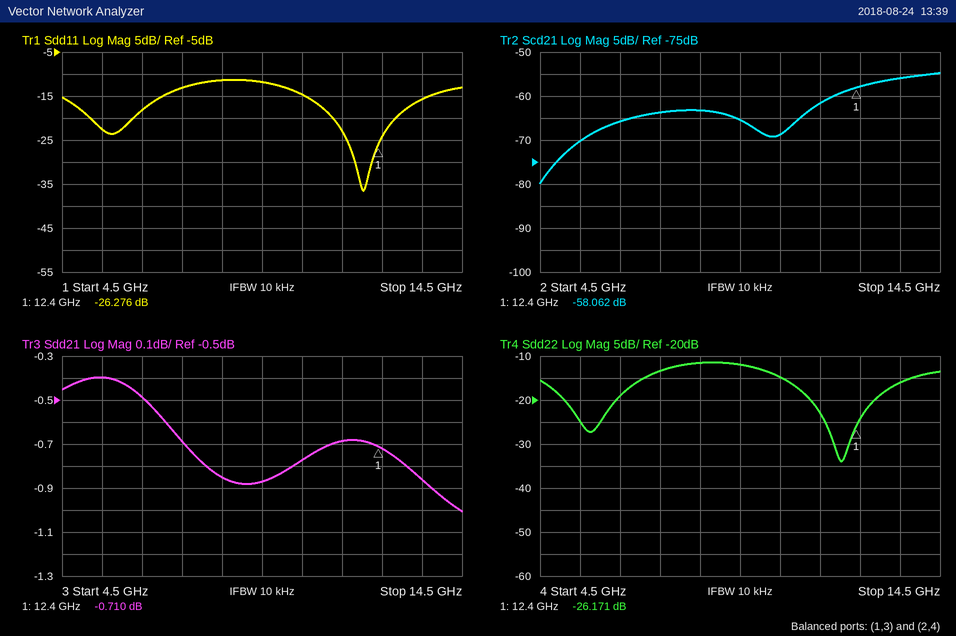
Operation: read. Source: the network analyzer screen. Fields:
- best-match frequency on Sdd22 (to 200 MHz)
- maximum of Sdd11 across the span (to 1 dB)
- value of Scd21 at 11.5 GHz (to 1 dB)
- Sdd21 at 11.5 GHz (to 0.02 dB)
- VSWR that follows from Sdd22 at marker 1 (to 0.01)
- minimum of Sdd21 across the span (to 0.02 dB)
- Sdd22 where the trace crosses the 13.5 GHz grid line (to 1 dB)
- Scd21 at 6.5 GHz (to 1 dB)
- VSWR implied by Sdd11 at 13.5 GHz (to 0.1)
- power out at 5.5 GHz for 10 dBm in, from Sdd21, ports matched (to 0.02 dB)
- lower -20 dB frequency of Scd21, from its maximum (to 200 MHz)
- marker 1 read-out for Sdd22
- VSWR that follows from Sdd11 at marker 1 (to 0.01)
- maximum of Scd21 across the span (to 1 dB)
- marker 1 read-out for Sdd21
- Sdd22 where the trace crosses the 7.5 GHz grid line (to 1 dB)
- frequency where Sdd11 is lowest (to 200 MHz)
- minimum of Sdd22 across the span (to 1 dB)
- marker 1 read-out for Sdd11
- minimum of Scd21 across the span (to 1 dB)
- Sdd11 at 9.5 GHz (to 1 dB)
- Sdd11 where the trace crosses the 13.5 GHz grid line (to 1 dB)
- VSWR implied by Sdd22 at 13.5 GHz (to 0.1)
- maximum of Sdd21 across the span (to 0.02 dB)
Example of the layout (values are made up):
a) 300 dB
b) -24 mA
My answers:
a) 12.0 GHz
b) -11 dB
c) -62 dB
d) -0.68 dB
e) 1.10
f) -1.00 dB
g) -16 dB
h) -66 dB
i) 1.4
j) 9.60 dBm
k) 5.0 GHz
l) -26.171 dB
m) 1.10
n) -55 dB
o) -0.710 dB
p) -13 dB
q) 12.0 GHz
r) -34 dB
s) -26.276 dB
t) -80 dB
u) -12 dB
v) -16 dB
w) 1.4
x) -0.40 dB
